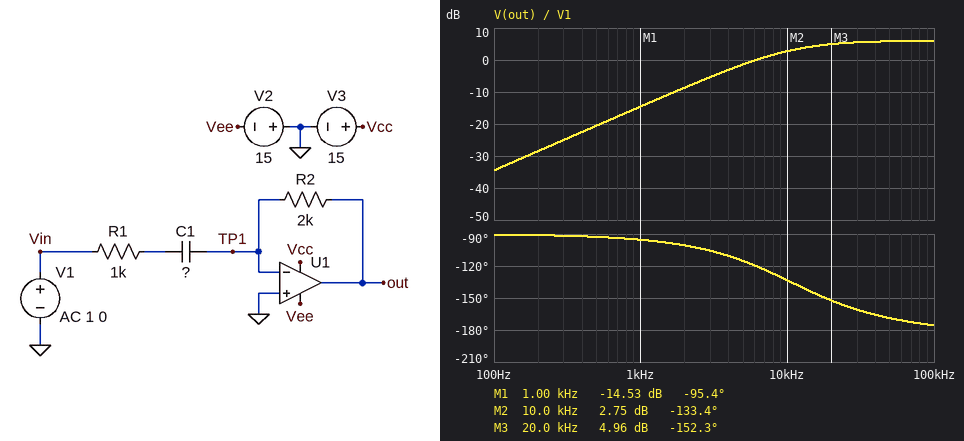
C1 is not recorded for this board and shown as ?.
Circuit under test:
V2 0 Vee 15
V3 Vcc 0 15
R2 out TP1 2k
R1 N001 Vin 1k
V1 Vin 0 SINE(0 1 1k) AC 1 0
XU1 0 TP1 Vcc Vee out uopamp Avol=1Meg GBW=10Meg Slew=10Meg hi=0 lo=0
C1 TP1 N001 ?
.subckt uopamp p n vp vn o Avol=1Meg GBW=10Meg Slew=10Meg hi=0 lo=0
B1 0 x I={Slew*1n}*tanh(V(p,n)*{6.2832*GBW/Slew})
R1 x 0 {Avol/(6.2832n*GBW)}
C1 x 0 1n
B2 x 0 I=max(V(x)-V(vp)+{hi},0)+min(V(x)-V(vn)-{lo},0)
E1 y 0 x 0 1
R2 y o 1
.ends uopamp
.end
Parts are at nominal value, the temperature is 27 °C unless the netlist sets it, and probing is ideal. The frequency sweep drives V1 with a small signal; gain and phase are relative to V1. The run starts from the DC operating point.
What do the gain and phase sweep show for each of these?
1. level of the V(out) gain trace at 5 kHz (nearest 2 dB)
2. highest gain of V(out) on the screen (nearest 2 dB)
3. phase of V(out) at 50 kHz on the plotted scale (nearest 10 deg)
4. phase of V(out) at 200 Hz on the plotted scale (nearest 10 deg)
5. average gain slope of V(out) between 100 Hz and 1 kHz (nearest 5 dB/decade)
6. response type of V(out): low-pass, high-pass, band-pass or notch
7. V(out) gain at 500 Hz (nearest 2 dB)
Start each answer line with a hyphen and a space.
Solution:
- -2 dB
- 6 dB
- -170 deg
- -90 deg
- 20 dB/decade
- high-pass
- -20 dB
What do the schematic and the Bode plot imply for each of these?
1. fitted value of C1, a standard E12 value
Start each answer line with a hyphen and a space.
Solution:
- 15 nF
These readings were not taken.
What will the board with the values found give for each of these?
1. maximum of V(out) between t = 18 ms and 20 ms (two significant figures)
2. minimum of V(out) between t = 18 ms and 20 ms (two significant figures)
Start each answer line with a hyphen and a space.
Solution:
- 190 mV
- -190 mV
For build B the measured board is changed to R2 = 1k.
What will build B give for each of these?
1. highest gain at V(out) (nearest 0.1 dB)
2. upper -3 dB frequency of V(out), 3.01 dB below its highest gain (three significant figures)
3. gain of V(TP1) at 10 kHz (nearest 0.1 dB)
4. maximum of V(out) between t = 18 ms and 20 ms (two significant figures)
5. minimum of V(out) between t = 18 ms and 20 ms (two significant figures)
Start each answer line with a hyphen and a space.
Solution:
- 0 dB
- 5.01 MHz
- -63.3 dB
- 94 mV
- -94 mV
